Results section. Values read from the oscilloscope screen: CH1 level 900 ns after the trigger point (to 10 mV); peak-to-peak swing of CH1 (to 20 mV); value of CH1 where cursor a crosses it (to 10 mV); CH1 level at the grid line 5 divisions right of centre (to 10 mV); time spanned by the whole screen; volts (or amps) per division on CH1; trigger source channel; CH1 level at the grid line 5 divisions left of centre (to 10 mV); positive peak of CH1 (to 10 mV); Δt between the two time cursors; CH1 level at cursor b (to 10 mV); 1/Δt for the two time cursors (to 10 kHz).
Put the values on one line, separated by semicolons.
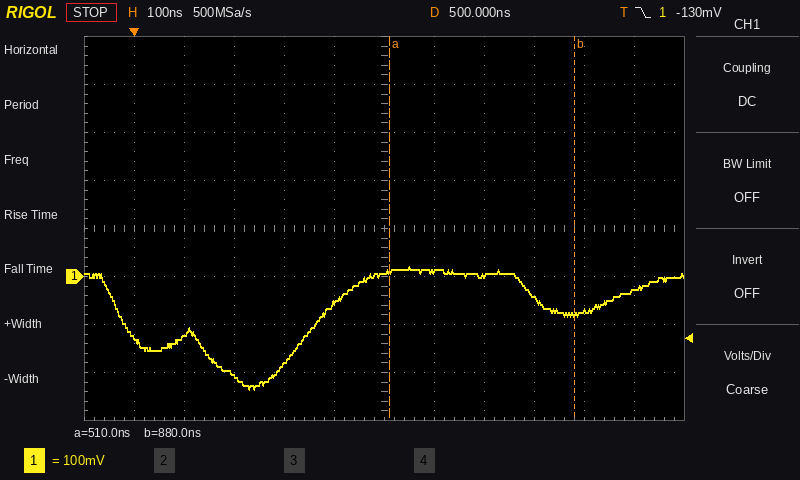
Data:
-70 mV; 260 mV; 10 mV; -30 mV; 1.2 µs; 100 mV; CH1; -130 mV; 20 mV; 370 ns; -80 mV; 2.70 MHz
